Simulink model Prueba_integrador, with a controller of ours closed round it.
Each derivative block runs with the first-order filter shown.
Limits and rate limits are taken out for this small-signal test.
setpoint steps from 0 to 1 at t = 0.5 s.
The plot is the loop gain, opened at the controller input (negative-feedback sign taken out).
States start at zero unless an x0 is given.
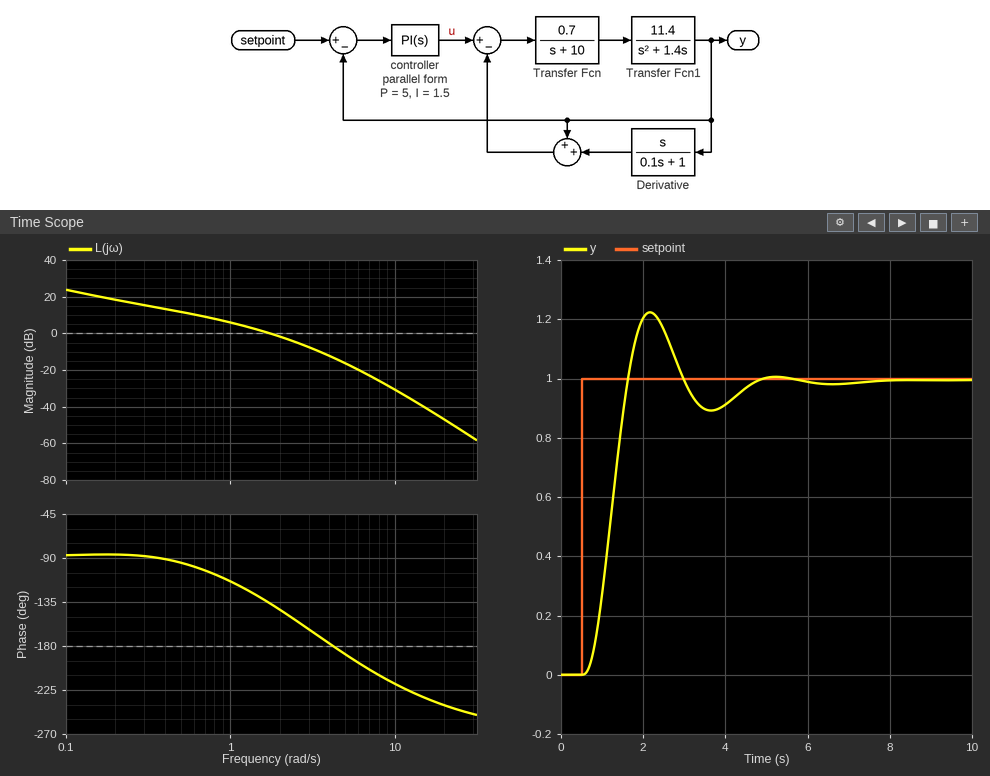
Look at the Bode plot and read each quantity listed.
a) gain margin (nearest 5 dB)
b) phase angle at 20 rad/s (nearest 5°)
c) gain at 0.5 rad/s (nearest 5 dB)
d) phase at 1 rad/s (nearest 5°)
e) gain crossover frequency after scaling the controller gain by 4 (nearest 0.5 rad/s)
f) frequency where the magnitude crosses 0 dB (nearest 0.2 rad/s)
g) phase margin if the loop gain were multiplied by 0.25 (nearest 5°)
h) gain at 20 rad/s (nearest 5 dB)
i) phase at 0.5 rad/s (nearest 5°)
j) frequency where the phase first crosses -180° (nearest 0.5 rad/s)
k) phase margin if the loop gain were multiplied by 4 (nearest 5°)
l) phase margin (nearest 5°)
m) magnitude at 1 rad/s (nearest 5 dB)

15 dB
-240°
10 dB
-115°
4.0 rad/s
1.8 rad/s
85°
-45 dB
-95°
4.0 rad/s
5°
45°
5 dB
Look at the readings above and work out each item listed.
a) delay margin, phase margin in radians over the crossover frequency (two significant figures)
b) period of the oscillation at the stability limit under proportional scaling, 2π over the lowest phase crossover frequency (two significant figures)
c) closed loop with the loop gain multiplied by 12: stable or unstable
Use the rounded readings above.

0.44 s
1.6 s
unstable
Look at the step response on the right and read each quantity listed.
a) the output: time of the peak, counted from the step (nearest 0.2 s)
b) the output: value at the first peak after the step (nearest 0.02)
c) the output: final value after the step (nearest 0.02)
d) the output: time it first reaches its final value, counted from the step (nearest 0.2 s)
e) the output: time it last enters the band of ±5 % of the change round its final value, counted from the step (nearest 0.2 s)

1.6 s
1.22
1.00
1.2 s
3.8 s
